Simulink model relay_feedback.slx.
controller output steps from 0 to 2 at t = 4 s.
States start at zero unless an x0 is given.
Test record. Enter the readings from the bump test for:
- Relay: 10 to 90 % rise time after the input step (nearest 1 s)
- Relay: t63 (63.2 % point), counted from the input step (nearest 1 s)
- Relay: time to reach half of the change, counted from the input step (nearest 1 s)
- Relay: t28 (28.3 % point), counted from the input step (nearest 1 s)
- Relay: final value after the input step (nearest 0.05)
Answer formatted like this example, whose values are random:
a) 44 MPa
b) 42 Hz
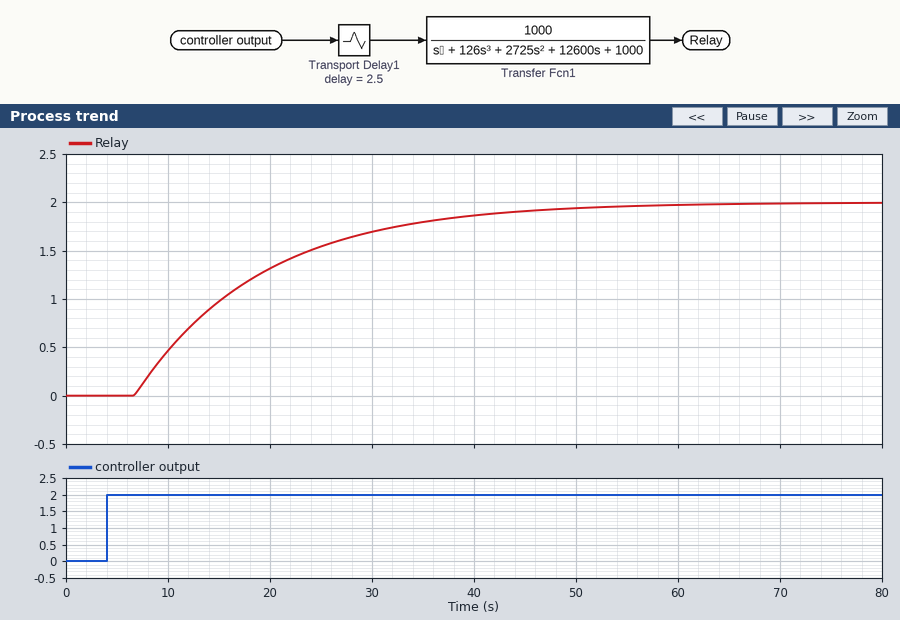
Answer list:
a) 27 s
b) 15 s
c) 11 s
d) 7 s
e) 2.00
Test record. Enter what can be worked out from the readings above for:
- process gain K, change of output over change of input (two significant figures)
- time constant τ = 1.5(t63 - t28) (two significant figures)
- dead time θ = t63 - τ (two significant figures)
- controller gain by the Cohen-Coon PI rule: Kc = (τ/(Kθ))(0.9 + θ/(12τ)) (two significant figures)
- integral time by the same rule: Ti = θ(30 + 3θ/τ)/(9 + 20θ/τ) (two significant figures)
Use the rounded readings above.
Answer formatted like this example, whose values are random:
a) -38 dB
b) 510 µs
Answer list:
a) 1.0
b) 12 s
c) 3.0 s
d) 3.7
e) 6.6 s
